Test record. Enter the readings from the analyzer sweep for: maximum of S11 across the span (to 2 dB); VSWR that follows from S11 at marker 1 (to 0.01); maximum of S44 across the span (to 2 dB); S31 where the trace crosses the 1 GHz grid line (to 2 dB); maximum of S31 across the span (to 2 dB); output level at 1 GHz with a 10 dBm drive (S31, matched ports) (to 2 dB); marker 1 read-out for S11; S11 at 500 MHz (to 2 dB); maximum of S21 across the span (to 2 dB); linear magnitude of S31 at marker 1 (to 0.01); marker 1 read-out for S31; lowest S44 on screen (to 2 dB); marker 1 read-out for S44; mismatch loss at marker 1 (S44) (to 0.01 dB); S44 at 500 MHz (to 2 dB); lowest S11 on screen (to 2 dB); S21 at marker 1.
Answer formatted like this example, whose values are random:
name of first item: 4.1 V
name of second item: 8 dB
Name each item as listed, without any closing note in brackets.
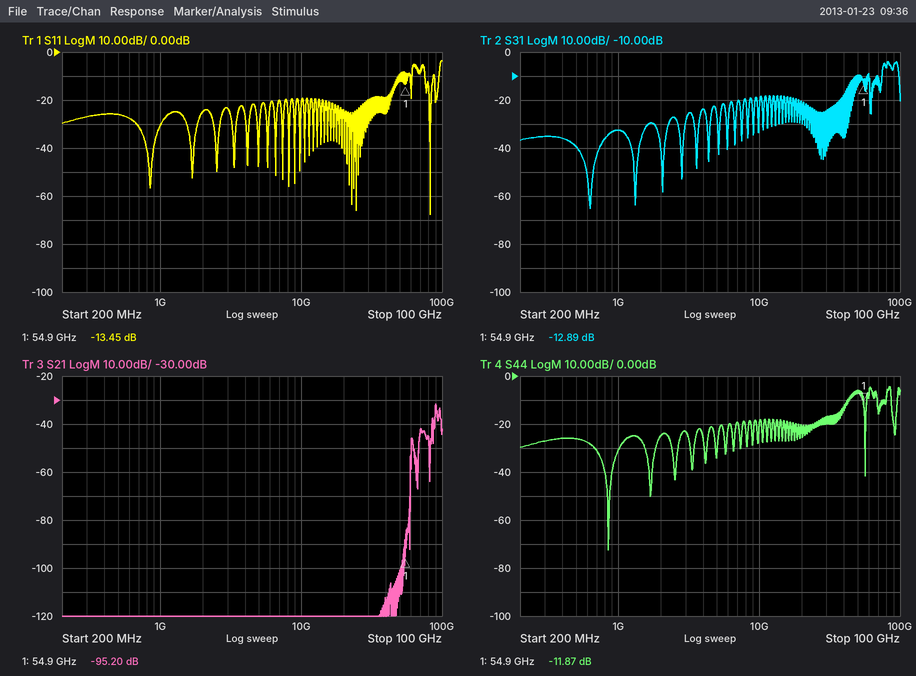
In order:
maximum of S11 across the span: -4 dB
VSWR that follows from S11 at marker 1: 1.54
maximum of S44 across the span: -4 dB
S31 where the trace crosses the 1 GHz grid line: -32 dB
maximum of S31 across the span: -4 dB
output level at 1 GHz with a 10 dBm drive (S31, matched ports): -22 dBm
marker 1 read-out for S11: -13.45 dB
S11 at 500 MHz: -26 dB
maximum of S21 across the span: -32 dB
linear magnitude of S31 at marker 1: 0.23
marker 1 read-out for S31: -12.89 dB
lowest S44 on screen: -72 dB
marker 1 read-out for S44: -11.87 dB
mismatch loss at marker 1 (S44): 0.29 dB
S44 at 500 MHz: -26 dB
lowest S11 on screen: -68 dB
S21 at marker 1: -95.20 dB
